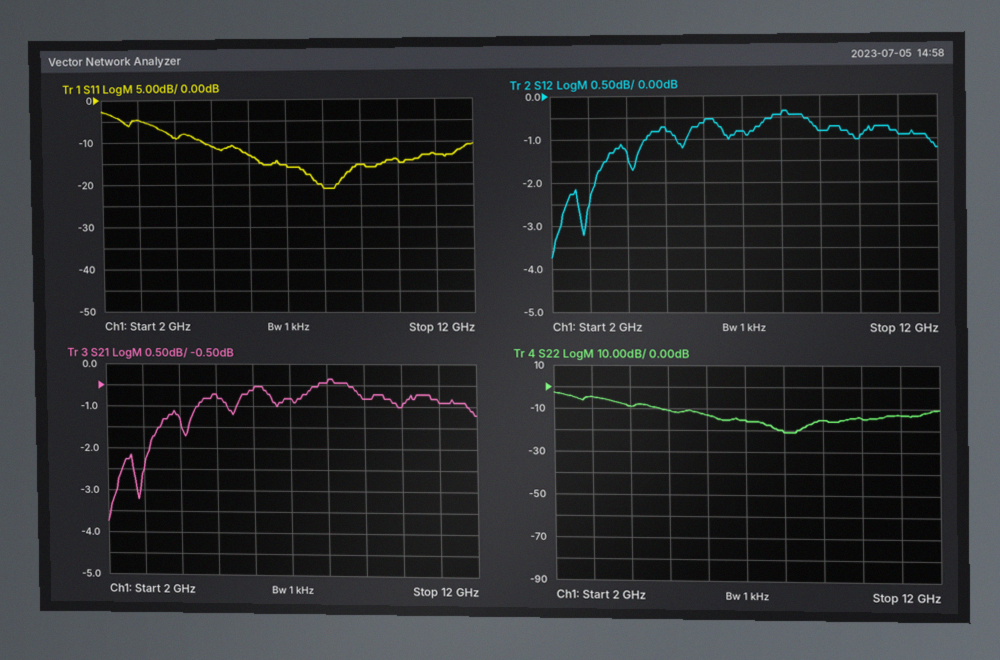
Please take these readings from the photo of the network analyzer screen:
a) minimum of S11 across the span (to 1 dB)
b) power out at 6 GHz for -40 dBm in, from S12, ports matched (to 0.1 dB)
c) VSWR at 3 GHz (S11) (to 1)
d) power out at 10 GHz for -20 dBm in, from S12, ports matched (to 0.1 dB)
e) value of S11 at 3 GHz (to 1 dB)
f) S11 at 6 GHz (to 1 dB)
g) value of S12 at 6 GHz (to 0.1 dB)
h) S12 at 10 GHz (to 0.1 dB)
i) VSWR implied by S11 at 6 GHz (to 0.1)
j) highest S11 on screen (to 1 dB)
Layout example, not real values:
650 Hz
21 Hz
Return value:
-21 dB
-40.6 dBm
4
-21.0 dBm
-5 dB
-13 dB
-0.6 dB
-1.0 dB
1.6
-3 dB
